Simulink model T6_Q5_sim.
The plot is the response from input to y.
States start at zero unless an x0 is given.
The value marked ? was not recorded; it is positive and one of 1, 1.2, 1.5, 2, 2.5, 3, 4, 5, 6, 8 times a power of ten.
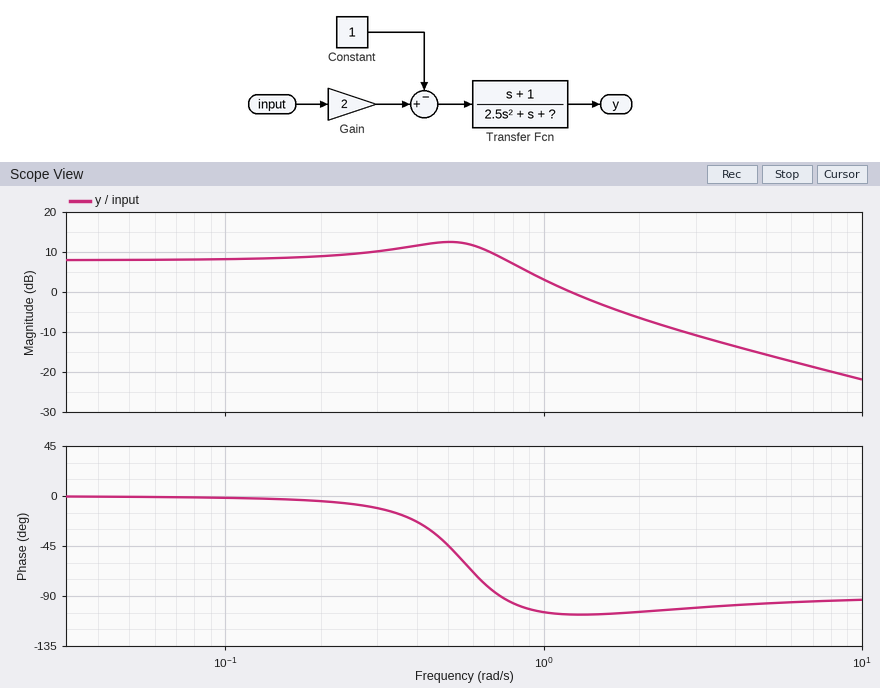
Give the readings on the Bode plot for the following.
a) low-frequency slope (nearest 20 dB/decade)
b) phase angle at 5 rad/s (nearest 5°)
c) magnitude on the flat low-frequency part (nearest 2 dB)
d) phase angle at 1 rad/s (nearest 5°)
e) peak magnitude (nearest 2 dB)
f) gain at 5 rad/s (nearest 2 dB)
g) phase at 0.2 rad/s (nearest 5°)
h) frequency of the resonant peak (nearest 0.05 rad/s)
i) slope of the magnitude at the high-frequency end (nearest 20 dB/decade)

0 dB/decade
-95°
8 dB
-105°
12 dB
-16 dB
-5°
0.50 rad/s
-20 dB/decade
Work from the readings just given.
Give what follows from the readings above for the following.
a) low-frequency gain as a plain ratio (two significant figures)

2.5
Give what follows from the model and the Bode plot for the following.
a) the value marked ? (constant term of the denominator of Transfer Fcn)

0.8
